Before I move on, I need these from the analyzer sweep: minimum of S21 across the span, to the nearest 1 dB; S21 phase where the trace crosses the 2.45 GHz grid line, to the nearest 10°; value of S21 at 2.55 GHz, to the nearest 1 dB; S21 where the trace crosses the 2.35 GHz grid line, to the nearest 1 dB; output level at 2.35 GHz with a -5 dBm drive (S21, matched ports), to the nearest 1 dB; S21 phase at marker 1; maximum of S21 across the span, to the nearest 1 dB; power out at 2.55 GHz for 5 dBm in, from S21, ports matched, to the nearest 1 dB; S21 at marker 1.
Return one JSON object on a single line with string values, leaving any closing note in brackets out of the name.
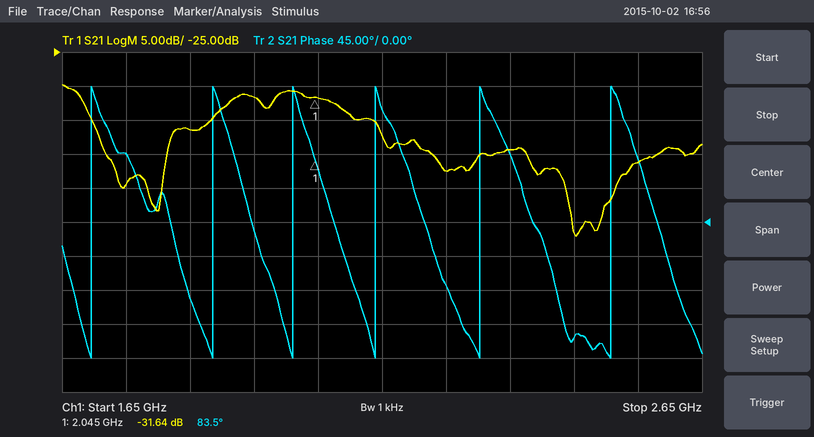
{"minimum of S21 across the span, to the nearest 1 dB": "-52 dB", "S21 phase where the trace crosses the 2.45 GHz grid line, to the nearest 10°": "-150°", "value of S21 at 2.55 GHz, to the nearest 1 dB": "-41 dB", "S21 where the trace crosses the 2.35 GHz grid line, to the nearest 1 dB": "-39 dB", "output level at 2.35 GHz with a -5 dBm drive (S21, matched ports), to the nearest 1 dB": "-44 dBm", "S21 phase at marker 1": "83.5°", "maximum of S21 across the span, to the nearest 1 dB": "-30 dB", "power out at 2.55 GHz for 5 dBm in, from S21, ports matched, to the nearest 1 dB": "-36 dBm", "S21 at marker 1": "-31.64 dB"}
